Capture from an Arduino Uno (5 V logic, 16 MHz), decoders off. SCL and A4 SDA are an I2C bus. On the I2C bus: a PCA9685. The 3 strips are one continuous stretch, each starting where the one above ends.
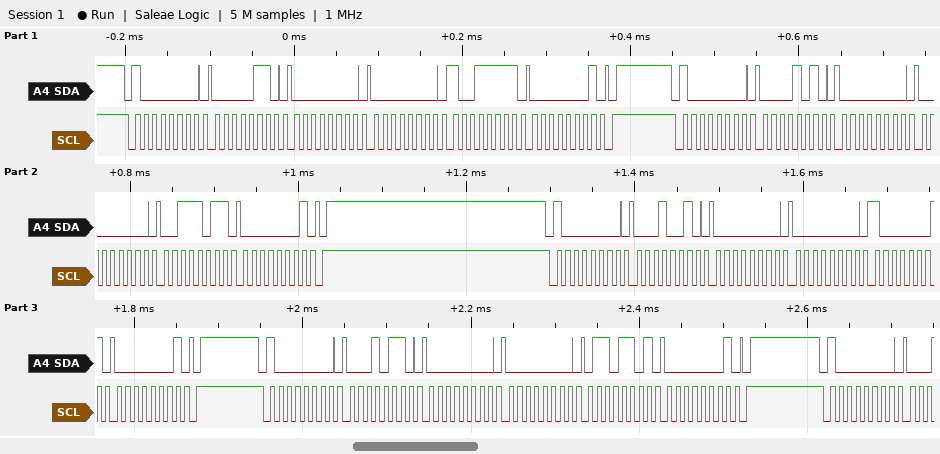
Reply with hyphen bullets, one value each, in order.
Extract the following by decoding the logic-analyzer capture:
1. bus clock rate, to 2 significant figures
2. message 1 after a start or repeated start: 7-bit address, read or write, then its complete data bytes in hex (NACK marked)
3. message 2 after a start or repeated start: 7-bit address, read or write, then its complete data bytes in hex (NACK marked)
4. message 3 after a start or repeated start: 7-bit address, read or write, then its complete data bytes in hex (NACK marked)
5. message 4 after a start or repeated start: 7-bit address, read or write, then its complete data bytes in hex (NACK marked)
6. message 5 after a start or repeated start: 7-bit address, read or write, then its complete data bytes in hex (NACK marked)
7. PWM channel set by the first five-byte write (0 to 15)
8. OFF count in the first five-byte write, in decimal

- 100 kHz
- 0x40 write: 06 00 00 9F 01
- 0x40 write: 0A 00 00 3B 01
- 0x40 write: 12 00 00 81 01
- 0x40 write: 16 00 00 6D 01
- 0x40 write
- 0
- 415
